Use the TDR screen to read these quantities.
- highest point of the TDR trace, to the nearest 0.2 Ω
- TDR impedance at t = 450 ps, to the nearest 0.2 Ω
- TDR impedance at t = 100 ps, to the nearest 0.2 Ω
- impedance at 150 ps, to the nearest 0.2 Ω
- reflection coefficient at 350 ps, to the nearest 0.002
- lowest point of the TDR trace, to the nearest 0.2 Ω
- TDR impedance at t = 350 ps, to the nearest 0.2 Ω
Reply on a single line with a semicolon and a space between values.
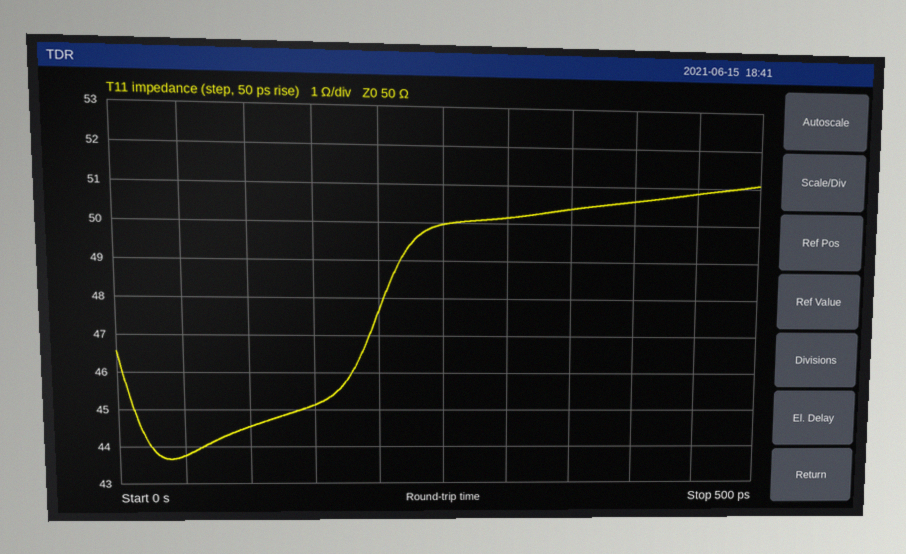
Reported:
51.0 Ω; 50.8 Ω; 44.6 Ω; 45.2 Ω; +0.004; 43.6 Ω; 50.4 Ω
